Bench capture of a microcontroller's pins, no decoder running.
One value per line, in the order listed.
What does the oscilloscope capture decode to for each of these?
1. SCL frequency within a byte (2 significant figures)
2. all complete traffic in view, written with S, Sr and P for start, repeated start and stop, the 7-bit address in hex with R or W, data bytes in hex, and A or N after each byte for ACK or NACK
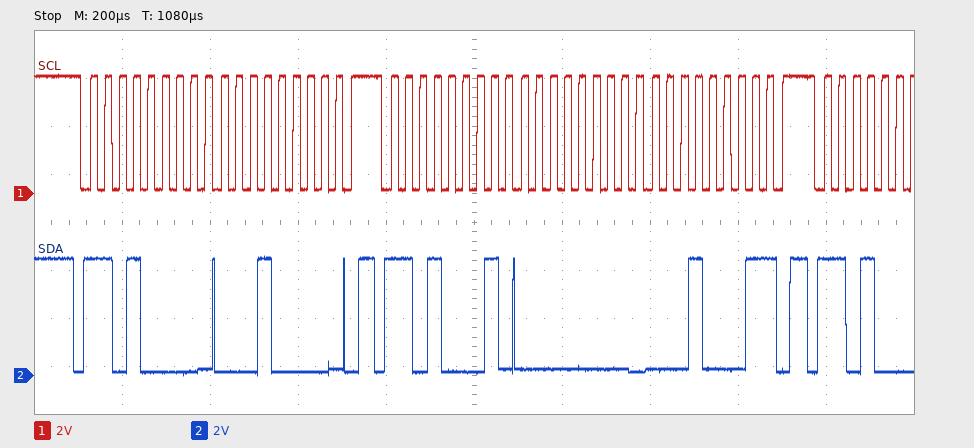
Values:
31 kHz
S 68W A 10 A P S 68R A 00 A 11 N P
